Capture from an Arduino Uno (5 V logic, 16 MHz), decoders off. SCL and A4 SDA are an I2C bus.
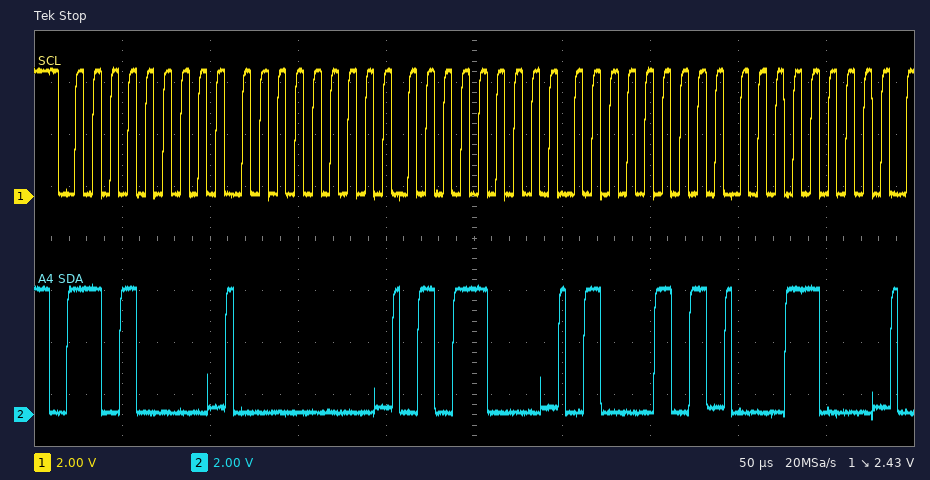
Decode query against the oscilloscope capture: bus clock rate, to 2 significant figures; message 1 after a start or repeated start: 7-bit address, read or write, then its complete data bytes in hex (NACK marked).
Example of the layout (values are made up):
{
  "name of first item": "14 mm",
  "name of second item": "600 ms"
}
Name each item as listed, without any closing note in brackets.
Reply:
{
  "bus clock rate, to 2 significant figures": "100 kHz",
  "message 1 after a start or repeated start: 7-bit address, read or write, then its complete data bytes in hex": "0x68 write: 00 58 45 18"
}
